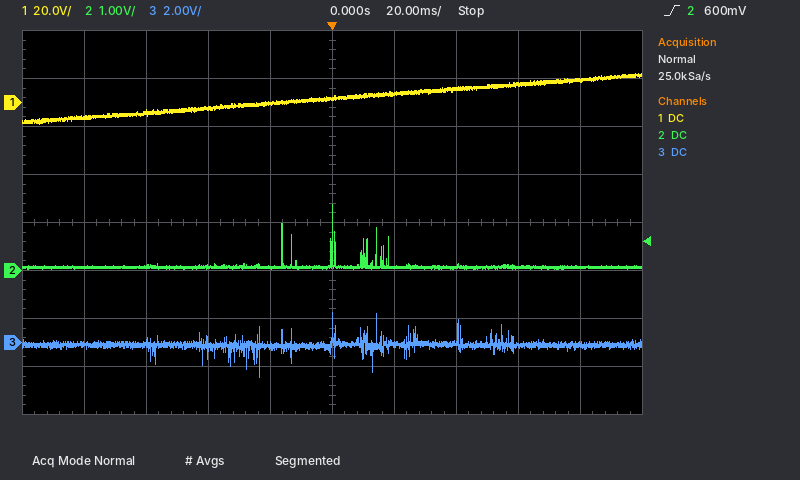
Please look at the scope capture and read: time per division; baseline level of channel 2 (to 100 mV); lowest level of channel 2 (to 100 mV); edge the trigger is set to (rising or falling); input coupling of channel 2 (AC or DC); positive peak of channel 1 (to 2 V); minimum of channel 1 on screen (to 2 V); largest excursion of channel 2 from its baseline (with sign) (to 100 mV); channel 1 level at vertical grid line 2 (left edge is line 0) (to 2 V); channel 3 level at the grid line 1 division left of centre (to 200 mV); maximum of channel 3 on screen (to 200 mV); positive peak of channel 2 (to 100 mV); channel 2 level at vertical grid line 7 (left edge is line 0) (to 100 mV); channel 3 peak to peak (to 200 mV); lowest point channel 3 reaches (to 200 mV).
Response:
20 ms
100 mV
0.0 V
rising
DC
12 V
-8 V
+1.3 V
-4 V
-200 mV
1.2 V
1.4 V
100 mV
2.6 V
-1.4 V
